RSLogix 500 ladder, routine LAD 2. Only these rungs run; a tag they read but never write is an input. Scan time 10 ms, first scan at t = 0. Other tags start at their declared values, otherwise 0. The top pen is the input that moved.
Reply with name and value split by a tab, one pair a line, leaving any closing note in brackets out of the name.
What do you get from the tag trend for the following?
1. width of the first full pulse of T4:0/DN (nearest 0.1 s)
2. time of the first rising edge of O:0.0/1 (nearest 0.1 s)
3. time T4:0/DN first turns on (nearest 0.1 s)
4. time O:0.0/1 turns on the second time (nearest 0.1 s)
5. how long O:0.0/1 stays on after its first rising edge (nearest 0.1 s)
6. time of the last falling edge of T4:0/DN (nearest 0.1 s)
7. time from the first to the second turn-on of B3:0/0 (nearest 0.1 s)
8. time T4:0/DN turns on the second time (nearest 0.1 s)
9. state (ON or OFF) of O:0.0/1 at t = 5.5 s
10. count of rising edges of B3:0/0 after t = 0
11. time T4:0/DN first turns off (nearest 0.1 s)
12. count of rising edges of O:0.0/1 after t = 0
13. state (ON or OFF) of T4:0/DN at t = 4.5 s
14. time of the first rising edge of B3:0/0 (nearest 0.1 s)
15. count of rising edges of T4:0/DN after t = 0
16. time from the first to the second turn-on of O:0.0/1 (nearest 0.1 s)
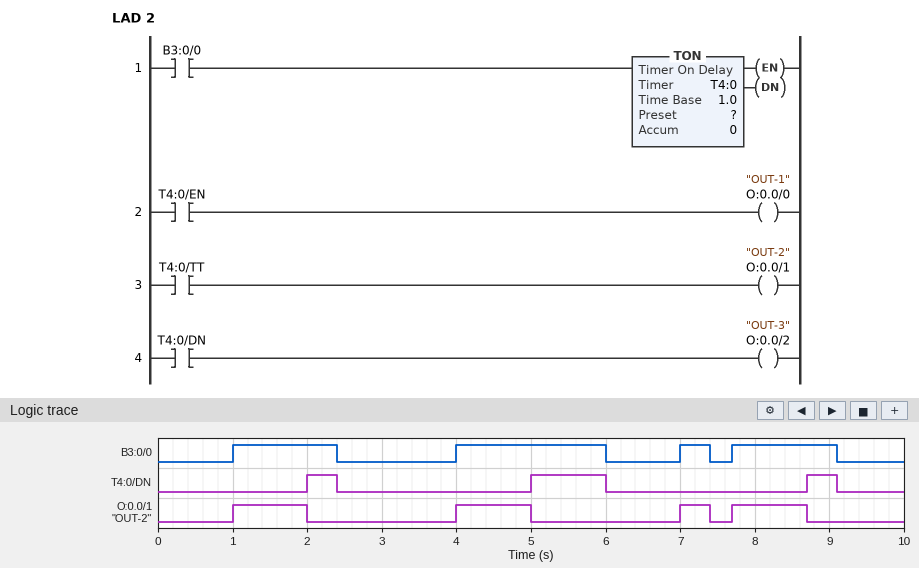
width of the first full pulse of T4:0/DN	0.4 s
time of the first rising edge of O:0.0/1	1.0 s
time T4:0/DN first turns on	2.0 s
time O:0.0/1 turns on the second time	4.0 s
how long O:0.0/1 stays on after its first rising edge	1.0 s
time of the last falling edge of T4:0/DN	9.1 s
time from the first to the second turn-on of B3:0/0	3.0 s
time T4:0/DN turns on the second time	5.0 s
state (ON or OFF) of O:0.0/1 at t = 5.5 s	OFF
count of rising edges of B3:0/0 after t = 0	4
time T4:0/DN first turns off	2.4 s
count of rising edges of O:0.0/1 after t = 0	4
state (ON or OFF) of T4:0/DN at t = 4.5 s	OFF
time of the first rising edge of B3:0/0	1.0 s
count of rising edges of T4:0/DN after t = 0	3
time from the first to the second turn-on of O:0.0/1	3.0 s
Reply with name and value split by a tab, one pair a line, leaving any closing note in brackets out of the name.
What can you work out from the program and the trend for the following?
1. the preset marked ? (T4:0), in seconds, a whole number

the preset marked ? (T4:0), in seconds, a whole number	1 s
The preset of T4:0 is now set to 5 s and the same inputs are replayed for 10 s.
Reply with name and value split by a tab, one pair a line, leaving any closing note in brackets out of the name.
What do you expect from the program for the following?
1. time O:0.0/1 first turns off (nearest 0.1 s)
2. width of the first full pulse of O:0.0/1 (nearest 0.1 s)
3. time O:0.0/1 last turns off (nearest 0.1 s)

time O:0.0/1 first turns off	2.4 s
width of the first full pulse of O:0.0/1	1.4 s
time O:0.0/1 last turns off	9.1 s
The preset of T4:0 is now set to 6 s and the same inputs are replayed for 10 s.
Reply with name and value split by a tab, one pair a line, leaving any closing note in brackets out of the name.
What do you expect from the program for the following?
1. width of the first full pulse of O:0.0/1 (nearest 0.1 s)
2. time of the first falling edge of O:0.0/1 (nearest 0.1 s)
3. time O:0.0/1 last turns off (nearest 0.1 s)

width of the first full pulse of O:0.0/1	1.4 s
time of the first falling edge of O:0.0/1	2.4 s
time O:0.0/1 last turns off	9.1 s
